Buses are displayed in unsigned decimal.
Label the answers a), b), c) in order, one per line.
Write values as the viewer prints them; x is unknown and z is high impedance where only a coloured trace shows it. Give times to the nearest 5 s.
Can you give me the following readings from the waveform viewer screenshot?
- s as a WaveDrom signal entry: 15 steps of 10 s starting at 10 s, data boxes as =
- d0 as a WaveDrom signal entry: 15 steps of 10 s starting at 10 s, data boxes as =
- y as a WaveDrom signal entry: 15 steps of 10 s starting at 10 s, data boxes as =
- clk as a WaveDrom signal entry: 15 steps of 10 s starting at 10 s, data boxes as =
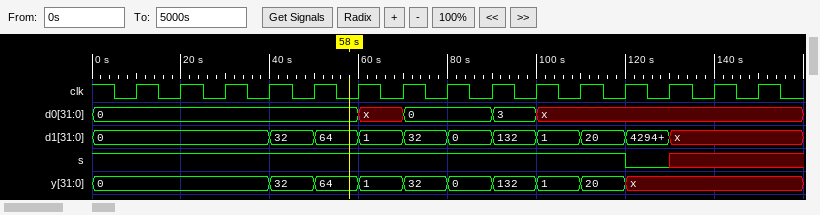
a) {name: 's', wave: '1..........0x..'}
b) {name: 'd0', wave: '=....x=.=x.....', data: '0 0 3'}
c) {name: 'y', wave: '=..========x...', data: '0 32 64 1 32 0 132 1 20'}
d) {name: 'clk', wave: 'p..............'}
